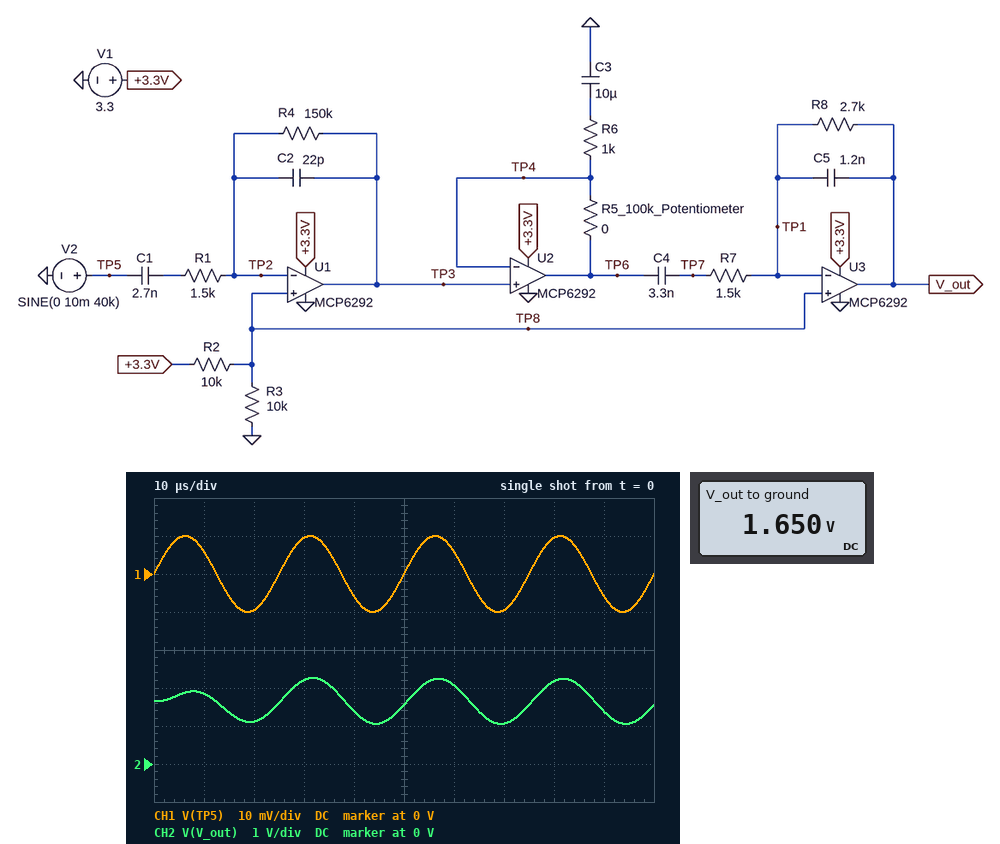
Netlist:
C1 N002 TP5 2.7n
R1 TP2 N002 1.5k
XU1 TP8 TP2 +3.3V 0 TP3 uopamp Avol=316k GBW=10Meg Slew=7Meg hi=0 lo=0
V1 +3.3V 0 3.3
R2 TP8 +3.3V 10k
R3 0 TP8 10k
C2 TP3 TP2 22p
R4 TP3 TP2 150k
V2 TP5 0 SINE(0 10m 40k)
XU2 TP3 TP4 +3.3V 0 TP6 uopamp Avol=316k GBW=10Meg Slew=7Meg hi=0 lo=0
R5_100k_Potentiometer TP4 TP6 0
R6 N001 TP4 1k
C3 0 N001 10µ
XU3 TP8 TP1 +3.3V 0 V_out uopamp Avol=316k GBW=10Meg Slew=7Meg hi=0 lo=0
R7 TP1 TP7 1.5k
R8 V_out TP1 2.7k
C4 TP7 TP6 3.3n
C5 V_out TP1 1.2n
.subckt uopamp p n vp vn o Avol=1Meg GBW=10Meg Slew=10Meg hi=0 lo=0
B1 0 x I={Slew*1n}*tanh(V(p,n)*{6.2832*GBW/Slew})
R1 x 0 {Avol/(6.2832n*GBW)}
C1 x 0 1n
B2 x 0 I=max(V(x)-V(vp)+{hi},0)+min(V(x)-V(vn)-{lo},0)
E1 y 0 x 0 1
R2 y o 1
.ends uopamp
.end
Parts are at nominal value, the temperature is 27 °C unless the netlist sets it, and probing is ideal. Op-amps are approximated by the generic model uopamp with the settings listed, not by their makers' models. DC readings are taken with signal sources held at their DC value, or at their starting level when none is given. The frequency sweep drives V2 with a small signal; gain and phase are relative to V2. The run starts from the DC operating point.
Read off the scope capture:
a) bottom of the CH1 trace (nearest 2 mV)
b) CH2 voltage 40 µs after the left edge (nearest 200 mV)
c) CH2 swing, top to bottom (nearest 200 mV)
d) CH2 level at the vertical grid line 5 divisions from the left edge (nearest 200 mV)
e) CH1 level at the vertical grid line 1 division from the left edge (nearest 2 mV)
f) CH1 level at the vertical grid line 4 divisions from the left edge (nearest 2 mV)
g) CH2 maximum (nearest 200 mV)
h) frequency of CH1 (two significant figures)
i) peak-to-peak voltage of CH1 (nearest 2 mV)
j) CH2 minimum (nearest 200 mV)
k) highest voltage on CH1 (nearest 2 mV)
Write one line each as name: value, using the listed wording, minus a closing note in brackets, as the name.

bottom of the CH1 trace: -10 mV
CH2 voltage 40 µs after the left edge: 1.4 V
CH2 swing, top to bottom: 1.2 V
CH2 level at the vertical grid line 5 divisions from the left edge: 1.6 V
CH1 level at the vertical grid line 1 division from the left edge: 6 mV
CH1 level at the vertical grid line 4 divisions from the left edge: -6 mV
CH2 maximum: 2.2 V
frequency of CH1: 40 kHz
peak-to-peak voltage of CH1: 20 mV
CH2 minimum: 1.0 V
highest voltage on CH1: 10 mV
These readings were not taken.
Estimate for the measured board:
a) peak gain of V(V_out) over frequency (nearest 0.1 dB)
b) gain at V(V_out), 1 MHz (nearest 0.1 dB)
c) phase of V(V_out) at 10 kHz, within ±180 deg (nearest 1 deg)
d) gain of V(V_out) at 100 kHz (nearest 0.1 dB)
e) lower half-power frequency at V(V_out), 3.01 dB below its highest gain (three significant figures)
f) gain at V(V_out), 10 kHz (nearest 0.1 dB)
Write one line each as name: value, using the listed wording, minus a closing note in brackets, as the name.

peak gain of V(V_out) over frequency: 35.5 dB
gain at V(V_out), 1 MHz: -11.0 dB
phase of V(V_out) at 10 kHz, within ±180 deg: 124 deg
gain of V(V_out) at 100 kHz: 27.3 dB
lower half-power frequency at V(V_out), 3.01 dB below its highest gain: 21.4 kHz
gain at V(V_out), 10 kHz: 22.2 dB
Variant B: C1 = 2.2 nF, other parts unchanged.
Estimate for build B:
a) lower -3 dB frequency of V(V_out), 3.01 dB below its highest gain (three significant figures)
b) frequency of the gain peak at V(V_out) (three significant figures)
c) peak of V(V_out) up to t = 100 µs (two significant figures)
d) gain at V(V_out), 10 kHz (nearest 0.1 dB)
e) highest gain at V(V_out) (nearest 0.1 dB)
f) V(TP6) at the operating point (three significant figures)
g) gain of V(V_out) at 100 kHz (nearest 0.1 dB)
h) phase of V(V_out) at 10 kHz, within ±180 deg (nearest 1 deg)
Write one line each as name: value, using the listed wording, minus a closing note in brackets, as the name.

lower -3 dB frequency of V(V_out), 3.01 dB below its highest gain: 22.7 kHz
frequency of the gain peak at V(V_out): 39.6 kHz
peak of V(V_out) up to t = 100 µs: 2.2 V
gain at V(V_out), 10 kHz: 20.5 dB
highest gain at V(V_out): 34.7 dB
V(TP6) at the operating point: 1.65 V
gain of V(V_out) at 100 kHz: 27.2 dB
phase of V(V_out) at 10 kHz, within ±180 deg: 127 deg
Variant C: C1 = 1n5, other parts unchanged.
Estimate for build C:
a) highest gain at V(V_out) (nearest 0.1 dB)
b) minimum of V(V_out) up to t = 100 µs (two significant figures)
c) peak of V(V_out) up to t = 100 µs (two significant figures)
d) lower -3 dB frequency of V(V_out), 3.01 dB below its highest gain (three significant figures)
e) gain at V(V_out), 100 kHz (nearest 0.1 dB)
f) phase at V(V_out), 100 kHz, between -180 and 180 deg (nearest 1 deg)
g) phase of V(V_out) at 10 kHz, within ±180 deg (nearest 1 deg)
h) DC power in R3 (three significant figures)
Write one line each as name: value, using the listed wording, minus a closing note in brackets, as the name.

highest gain at V(V_out): 32.8 dB
minimum of V(V_out) up to t = 100 µs: 1.2 V
peak of V(V_out) up to t = 100 µs: 2.1 V
lower -3 dB frequency of V(V_out), 3.01 dB below its highest gain: 25.1 kHz
gain at V(V_out), 100 kHz: 26.8 dB
phase at V(V_out), 100 kHz, between -180 and 180 deg: -92 deg
phase of V(V_out) at 10 kHz, within ±180 deg: 131 deg
DC power in R3: 272 µW
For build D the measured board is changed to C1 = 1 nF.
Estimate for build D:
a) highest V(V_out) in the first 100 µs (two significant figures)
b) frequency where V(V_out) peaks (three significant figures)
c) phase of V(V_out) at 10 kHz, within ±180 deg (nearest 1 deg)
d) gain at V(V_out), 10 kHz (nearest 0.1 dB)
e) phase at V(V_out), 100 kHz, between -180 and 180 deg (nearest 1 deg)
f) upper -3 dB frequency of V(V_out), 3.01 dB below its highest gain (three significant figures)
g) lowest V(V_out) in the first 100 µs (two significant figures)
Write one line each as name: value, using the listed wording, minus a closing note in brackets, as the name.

highest V(V_out) in the first 100 µs: 2.0 V
frequency where V(V_out) peaks: 49.5 kHz
phase of V(V_out) at 10 kHz, within ±180 deg: 134 deg
gain at V(V_out), 10 kHz: 13.7 dB
phase at V(V_out), 100 kHz, between -180 and 180 deg: -80 deg
upper -3 dB frequency of V(V_out), 3.01 dB below its highest gain: 88.5 kHz
lowest V(V_out) in the first 100 µs: 1.3 V
